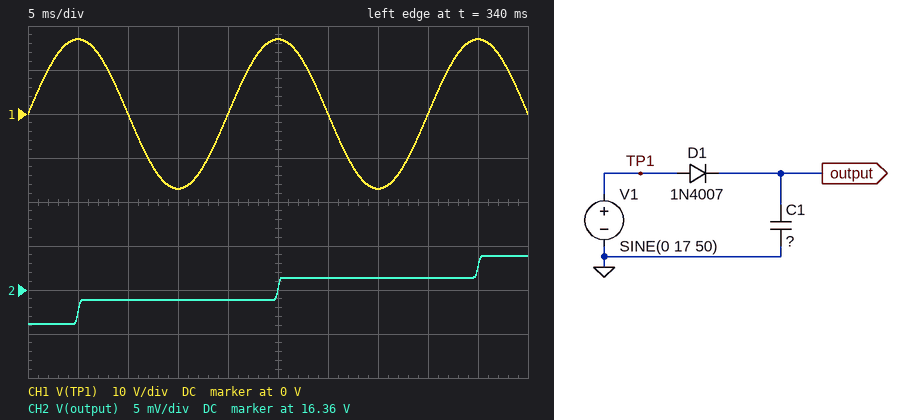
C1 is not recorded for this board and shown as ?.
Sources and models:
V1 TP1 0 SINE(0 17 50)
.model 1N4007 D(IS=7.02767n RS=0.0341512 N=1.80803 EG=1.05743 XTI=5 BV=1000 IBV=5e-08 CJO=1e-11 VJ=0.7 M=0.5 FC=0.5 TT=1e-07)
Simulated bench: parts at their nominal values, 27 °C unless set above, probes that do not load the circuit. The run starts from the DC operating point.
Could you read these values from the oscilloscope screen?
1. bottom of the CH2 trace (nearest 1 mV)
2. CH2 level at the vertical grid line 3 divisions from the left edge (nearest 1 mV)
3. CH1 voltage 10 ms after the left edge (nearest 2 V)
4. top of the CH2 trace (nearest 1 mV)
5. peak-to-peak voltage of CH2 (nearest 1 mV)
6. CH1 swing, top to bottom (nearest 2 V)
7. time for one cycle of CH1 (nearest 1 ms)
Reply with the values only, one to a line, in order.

16.356 V
16.359 V
0 V
16.364 V
8 mV
34 V
20 ms
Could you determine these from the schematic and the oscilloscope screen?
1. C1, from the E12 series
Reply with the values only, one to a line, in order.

1 mF
